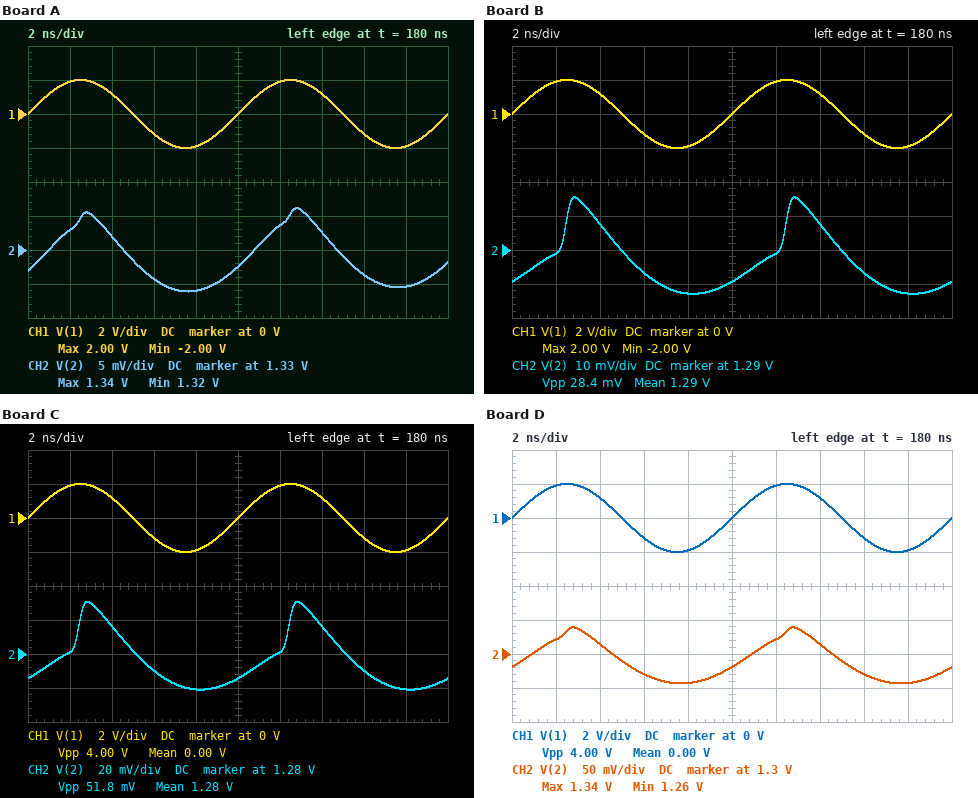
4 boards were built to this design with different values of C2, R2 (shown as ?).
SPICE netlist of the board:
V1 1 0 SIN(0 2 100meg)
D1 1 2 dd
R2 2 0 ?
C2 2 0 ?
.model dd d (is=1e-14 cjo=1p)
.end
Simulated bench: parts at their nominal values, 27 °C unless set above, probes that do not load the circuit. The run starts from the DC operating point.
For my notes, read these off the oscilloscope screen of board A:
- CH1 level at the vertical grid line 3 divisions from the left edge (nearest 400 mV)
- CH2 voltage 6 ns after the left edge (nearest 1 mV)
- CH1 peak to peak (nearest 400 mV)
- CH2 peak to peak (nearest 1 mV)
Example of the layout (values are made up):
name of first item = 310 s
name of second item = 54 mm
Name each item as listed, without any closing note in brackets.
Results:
CH1 level at the vertical grid line 3 divisions from the left edge = -1.2 V
CH2 voltage 6 ns after the left edge = 1.326 V
CH1 peak to peak = 4.0 V
CH2 peak to peak = 12 mV
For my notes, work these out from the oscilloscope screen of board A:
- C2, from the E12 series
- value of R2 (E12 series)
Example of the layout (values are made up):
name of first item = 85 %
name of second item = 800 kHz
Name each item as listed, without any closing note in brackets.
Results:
C2, from the E12 series = 270 pF
value of R2 = 27 kΩ
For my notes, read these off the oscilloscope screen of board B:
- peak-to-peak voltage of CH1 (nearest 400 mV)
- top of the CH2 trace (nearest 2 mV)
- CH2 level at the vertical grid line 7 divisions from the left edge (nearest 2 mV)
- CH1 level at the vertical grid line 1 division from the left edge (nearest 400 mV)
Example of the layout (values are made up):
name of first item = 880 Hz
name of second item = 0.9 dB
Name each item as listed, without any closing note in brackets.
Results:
peak-to-peak voltage of CH1 = 4.0 V
top of the CH2 trace = 1.306 V
CH2 level at the vertical grid line 7 divisions from the left edge = 1.298 V
CH1 level at the vertical grid line 1 division from the left edge = 2.0 V
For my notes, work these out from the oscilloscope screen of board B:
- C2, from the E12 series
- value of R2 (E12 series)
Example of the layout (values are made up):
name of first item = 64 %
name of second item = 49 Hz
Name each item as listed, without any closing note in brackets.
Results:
C2, from the E12 series = 150 pF
value of R2 = 4.7 kΩ
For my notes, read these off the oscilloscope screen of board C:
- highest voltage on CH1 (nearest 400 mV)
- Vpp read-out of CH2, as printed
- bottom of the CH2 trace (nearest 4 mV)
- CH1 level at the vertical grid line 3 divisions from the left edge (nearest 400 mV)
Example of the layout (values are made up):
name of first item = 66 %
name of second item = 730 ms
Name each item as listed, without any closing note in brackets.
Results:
highest voltage on CH1 = 2.0 V
Vpp read-out of CH2, as printed = 51.8 mV
bottom of the CH2 trace = 1.260 V
CH1 level at the vertical grid line 3 divisions from the left edge = -1.2 V
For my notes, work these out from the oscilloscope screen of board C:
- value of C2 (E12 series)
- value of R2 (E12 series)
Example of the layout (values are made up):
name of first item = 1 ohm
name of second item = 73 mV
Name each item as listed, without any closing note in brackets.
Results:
value of C2 = 82 pF
value of R2 = 4.7 kΩ
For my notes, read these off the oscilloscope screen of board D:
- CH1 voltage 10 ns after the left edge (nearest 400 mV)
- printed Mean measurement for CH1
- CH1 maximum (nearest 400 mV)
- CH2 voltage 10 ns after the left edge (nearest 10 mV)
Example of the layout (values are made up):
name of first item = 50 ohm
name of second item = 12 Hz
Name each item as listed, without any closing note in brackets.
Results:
CH1 voltage 10 ns after the left edge = 0 V
printed Mean measurement for CH1 = 0.00 V
CH1 maximum = 2.0 V
CH2 voltage 10 ns after the left edge = 1.28 V
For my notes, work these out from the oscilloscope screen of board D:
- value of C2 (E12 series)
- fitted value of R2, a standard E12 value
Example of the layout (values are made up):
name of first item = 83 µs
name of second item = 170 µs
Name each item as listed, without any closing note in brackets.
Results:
value of C2 = 39 pF
fitted value of R2, a standard E12 value = 18 kΩ
